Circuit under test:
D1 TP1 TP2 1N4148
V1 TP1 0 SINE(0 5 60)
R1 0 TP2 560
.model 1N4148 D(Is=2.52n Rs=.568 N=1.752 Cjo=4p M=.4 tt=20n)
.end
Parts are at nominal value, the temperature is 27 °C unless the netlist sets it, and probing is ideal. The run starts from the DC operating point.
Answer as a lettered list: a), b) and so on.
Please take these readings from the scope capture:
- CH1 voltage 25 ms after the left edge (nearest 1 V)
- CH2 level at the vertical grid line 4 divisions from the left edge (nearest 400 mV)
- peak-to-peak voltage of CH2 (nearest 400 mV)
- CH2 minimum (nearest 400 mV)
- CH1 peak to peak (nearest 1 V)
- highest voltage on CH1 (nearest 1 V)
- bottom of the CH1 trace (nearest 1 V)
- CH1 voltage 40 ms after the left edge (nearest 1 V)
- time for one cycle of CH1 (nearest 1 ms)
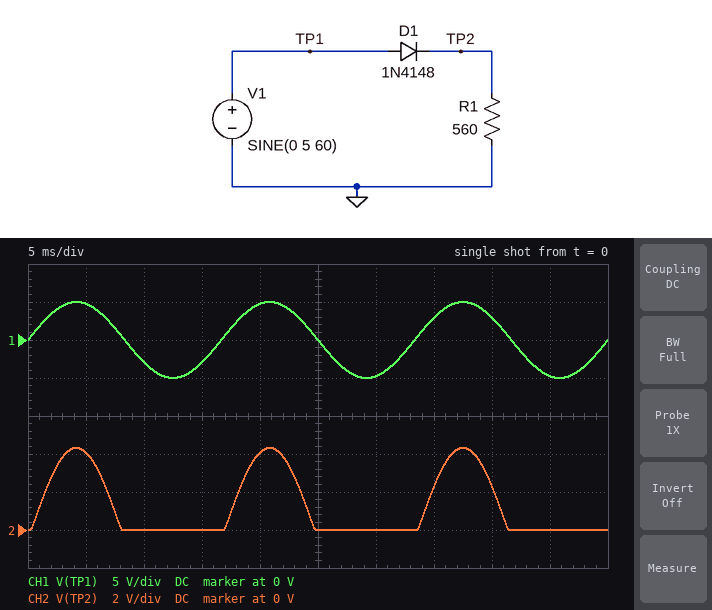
a) 0 V
b) 4.0 V
c) 4.4 V
d) 0 V
e) 10 V
f) 5 V
g) -5 V
h) 3 V
i) 17 ms
